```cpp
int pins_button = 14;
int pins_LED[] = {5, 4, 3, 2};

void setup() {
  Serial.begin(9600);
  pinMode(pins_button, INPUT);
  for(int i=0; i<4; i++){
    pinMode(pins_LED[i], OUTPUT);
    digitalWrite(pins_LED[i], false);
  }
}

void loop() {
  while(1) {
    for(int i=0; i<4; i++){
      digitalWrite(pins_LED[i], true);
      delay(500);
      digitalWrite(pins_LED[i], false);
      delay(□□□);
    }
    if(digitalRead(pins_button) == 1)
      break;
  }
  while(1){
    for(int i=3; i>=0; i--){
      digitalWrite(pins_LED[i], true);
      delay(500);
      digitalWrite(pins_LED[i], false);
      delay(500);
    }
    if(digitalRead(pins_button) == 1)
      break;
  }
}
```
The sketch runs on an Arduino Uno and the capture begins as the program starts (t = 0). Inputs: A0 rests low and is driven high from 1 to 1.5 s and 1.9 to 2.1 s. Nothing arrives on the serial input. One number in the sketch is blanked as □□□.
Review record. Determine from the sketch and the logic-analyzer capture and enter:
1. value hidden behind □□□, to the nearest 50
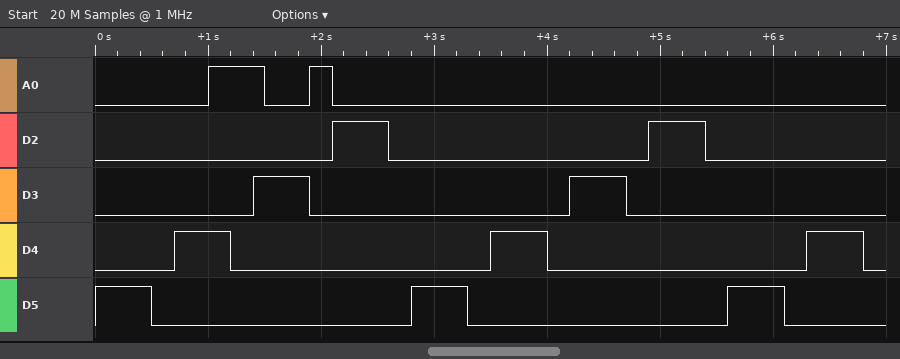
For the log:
200
